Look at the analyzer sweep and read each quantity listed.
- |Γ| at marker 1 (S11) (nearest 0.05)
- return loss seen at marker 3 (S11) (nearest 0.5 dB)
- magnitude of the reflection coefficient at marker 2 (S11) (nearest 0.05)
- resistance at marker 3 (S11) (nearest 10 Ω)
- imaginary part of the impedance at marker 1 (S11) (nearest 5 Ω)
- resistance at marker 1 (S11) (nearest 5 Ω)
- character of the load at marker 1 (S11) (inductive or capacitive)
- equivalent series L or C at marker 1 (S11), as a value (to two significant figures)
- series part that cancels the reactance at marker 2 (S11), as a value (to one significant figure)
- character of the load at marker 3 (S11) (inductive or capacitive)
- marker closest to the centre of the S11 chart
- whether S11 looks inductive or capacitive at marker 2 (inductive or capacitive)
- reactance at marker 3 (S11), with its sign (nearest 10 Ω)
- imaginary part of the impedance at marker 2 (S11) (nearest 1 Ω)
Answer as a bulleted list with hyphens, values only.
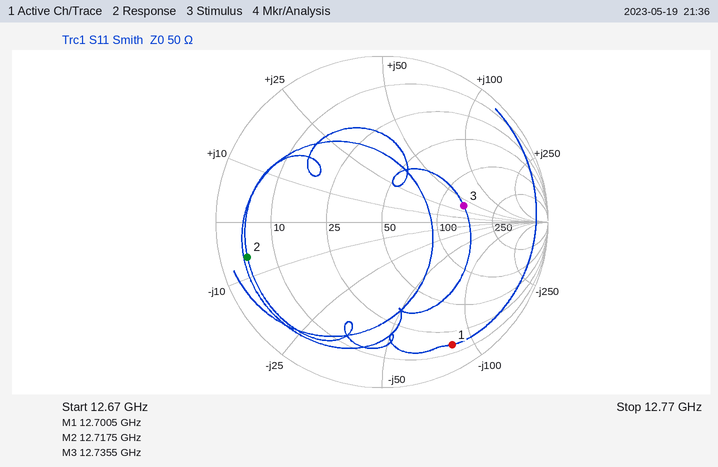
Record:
- 0.85
- 6.0 dB
- 0.85
- 140 Ω
- -85 Ω
- 15 Ω
- capacitive
- 150 fF
- 80 pH
- inductive
- marker 3
- capacitive
- +40 Ω
- -6 Ω
